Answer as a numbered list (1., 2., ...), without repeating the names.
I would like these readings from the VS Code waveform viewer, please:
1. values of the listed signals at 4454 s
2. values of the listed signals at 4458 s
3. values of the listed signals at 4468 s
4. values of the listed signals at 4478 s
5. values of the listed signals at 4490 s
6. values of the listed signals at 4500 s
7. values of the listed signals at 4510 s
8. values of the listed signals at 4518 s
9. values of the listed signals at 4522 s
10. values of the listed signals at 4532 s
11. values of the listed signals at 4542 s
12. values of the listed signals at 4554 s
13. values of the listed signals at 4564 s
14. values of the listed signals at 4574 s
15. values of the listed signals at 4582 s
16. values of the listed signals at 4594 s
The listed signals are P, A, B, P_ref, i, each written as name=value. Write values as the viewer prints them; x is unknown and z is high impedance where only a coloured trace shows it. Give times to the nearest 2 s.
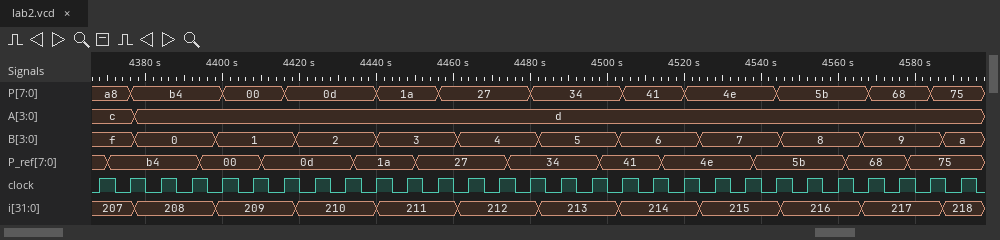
1. P=1a, A=d, B=3, P_ref=27, i=211
2. P=27, A=d, B=3, P_ref=27, i=211
3. P=27, A=d, B=4, P_ref=27, i=212
4. P=27, A=d, B=4, P_ref=34, i=212
5. P=34, A=d, B=5, P_ref=34, i=213
6. P=34, A=d, B=5, P_ref=41, i=213
7. P=41, A=d, B=6, P_ref=41, i=214
8. P=41, A=d, B=6, P_ref=4e, i=214
9. P=4e, A=d, B=6, P_ref=4e, i=214
10. P=4e, A=d, B=7, P_ref=4e, i=215
11. P=4e, A=d, B=7, P_ref=5b, i=215
12. P=5b, A=d, B=8, P_ref=5b, i=216
13. P=5b, A=d, B=8, P_ref=68, i=216
14. P=68, A=d, B=9, P_ref=68, i=217
15. P=68, A=d, B=9, P_ref=75, i=217
16. P=75, A=d, B=a, P_ref=75, i=218
